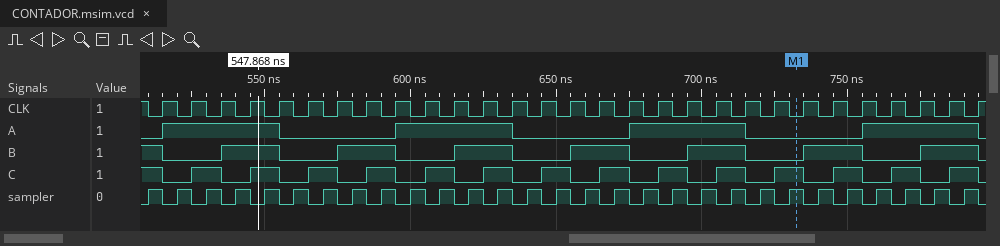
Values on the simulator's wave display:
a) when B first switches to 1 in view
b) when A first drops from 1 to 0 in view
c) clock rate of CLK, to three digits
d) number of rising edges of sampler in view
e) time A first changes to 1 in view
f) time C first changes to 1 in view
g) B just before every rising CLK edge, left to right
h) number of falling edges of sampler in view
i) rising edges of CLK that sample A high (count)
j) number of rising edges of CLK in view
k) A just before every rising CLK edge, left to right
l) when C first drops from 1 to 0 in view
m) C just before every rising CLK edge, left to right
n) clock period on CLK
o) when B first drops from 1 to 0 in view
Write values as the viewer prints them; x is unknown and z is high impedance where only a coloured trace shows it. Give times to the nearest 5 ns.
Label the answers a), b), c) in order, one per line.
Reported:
a) 535 ns
b) 555 ns
c) 100 MHz
d) 29
e) 515 ns
f) 525 ns
g) 1 0 0 1 1 0 0 1 1 0 0 1 1 0 0 1 1 0 0 1 1 0 0 1 1 0 0 1 1
h) 29
i) 16
j) 29
k) 0 1 1 1 1 0 0 0 0 1 1 1 1 0 0 0 0 1 1 1 1 0 0 0 0 1 1 1 1
l) 515 ns
m) 1 0 1 0 1 0 1 0 1 0 1 0 1 0 1 0 1 0 1 0 1 0 1 0 1 0 1 0 1
n) 10 ns
o) 515 ns
